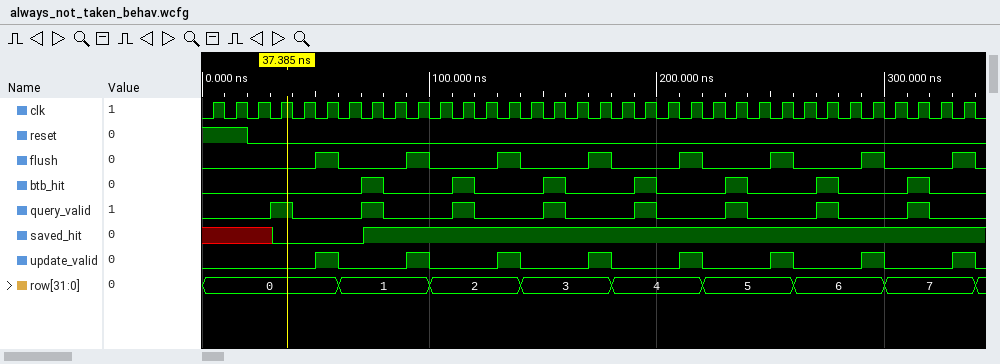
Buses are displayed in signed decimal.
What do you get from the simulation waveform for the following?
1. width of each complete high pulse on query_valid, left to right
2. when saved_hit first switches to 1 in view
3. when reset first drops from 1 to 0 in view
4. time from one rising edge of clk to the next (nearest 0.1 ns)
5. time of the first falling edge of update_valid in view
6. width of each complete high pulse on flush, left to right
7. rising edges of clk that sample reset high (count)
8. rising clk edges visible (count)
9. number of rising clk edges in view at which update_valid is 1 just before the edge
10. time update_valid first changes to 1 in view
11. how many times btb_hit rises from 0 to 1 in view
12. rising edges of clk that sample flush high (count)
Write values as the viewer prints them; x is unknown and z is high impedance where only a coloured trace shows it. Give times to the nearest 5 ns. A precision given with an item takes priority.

10 ns, 10 ns, 10 ns, 10 ns, 10 ns, 10 ns, 10 ns, 10 ns
70 ns
20 ns
10 ns
60 ns
10 ns, 10 ns, 10 ns, 10 ns, 10 ns, 10 ns, 10 ns, 10 ns
2
34
8
50 ns
7
8
